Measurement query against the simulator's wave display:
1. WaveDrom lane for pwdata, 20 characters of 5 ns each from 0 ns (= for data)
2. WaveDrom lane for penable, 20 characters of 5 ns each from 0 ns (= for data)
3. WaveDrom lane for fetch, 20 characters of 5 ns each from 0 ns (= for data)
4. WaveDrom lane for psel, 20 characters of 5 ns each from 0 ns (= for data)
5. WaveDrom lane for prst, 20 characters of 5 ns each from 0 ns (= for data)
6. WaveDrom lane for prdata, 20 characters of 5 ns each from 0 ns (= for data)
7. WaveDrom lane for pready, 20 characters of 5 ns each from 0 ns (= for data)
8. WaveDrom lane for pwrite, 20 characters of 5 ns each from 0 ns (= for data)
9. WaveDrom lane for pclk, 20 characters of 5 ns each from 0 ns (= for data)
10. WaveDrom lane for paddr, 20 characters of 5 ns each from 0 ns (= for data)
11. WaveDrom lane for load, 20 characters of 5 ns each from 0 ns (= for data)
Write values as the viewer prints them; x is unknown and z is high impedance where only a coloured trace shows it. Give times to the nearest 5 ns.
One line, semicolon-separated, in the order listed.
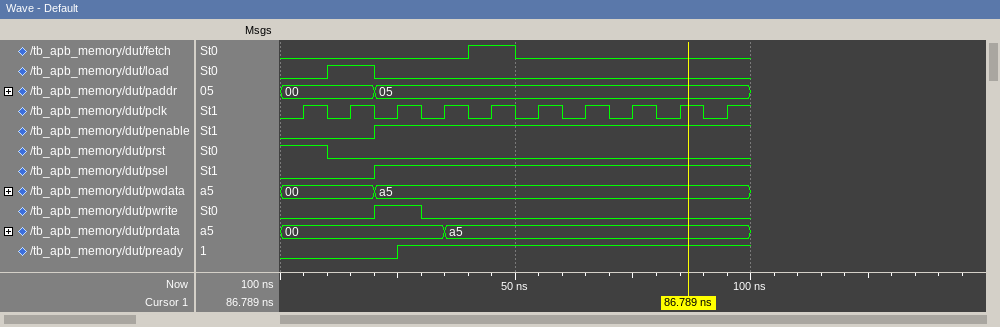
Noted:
{name: 'pwdata', wave: '=...=...............', data: '00 a5'}; {name: 'penable', wave: '0...1...............'}; {name: 'fetch', wave: '0.......1.0.........'}; {name: 'psel', wave: '0...1...............'}; {name: 'prst', wave: '1.0.................'}; {name: 'prdata', wave: '=......=............', data: '00 a5'}; {name: 'pready', wave: '0....1..............'}; {name: 'pwrite', wave: '0...1.0.............'}; {name: 'pclk', wave: '01010101010101010101'}; {name: 'paddr', wave: '=...=...............', data: '00 05'}; {name: 'load', wave: '0.1.0...............'}
